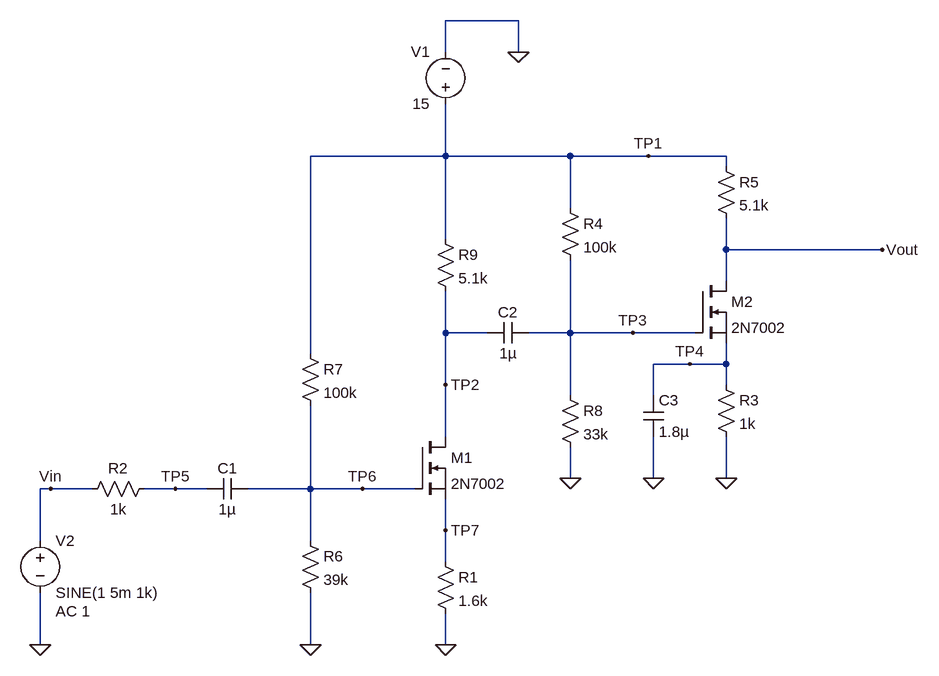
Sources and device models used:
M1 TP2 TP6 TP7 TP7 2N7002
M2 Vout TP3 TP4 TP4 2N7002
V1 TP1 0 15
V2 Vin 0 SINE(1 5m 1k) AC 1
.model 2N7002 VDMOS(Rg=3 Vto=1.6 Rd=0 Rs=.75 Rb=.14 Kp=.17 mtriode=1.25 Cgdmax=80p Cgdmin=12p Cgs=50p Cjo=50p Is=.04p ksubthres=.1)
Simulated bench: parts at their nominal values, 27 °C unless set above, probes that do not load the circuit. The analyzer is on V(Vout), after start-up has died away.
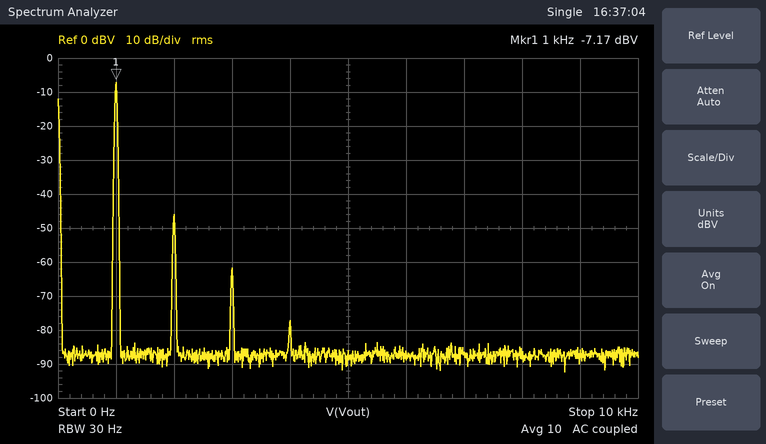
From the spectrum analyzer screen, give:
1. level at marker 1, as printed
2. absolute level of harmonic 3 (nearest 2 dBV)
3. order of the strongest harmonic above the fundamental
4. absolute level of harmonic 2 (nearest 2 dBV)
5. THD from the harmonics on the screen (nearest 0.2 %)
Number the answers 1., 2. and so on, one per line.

1. -7.17 dBV
2. -62 dBV
3. 2
4. -46 dBV
5. 1.2 %
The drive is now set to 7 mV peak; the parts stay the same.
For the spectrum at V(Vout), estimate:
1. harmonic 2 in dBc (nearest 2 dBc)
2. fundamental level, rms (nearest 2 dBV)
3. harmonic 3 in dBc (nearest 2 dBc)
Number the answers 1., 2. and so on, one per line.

1. -36 dBc
2. -4 dBV
3. -48 dBc
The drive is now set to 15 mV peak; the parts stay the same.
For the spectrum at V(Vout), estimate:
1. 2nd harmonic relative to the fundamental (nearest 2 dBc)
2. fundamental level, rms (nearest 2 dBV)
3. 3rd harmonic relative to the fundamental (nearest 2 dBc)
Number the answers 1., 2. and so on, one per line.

1. -28 dBc
2. 2 dBV
3. -36 dBc
